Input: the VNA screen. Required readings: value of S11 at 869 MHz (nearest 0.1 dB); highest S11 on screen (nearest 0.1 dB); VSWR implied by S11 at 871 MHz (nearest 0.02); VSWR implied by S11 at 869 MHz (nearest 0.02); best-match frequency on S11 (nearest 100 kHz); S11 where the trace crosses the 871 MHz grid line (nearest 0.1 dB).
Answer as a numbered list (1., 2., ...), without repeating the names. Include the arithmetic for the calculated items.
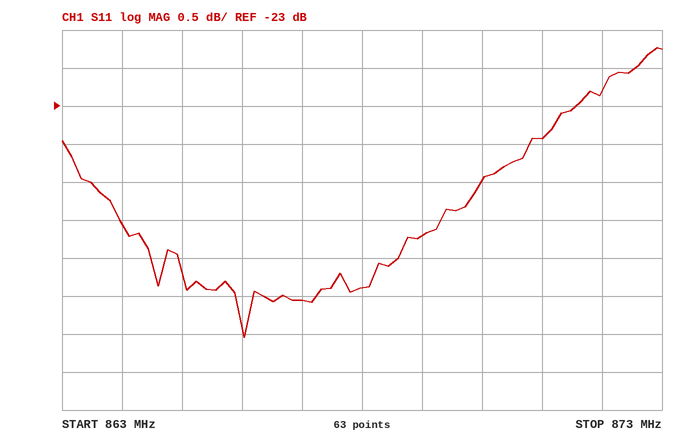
1. -24.7 dB
2. -22.2 dB
3. |Γ| = 10^(-23.4/20) = 0.0676; VSWR = (1 + 0.0676)/(1 − 0.0676) ≈ 1.15, so 1.14 to the nearest 0.02
4. |Γ| = 10^(-24.7/20) = 0.0582; VSWR = (1 + 0.0582)/(1 − 0.0582) ≈ 1.12
5. 866.0 MHz
6. -23.4 dB
